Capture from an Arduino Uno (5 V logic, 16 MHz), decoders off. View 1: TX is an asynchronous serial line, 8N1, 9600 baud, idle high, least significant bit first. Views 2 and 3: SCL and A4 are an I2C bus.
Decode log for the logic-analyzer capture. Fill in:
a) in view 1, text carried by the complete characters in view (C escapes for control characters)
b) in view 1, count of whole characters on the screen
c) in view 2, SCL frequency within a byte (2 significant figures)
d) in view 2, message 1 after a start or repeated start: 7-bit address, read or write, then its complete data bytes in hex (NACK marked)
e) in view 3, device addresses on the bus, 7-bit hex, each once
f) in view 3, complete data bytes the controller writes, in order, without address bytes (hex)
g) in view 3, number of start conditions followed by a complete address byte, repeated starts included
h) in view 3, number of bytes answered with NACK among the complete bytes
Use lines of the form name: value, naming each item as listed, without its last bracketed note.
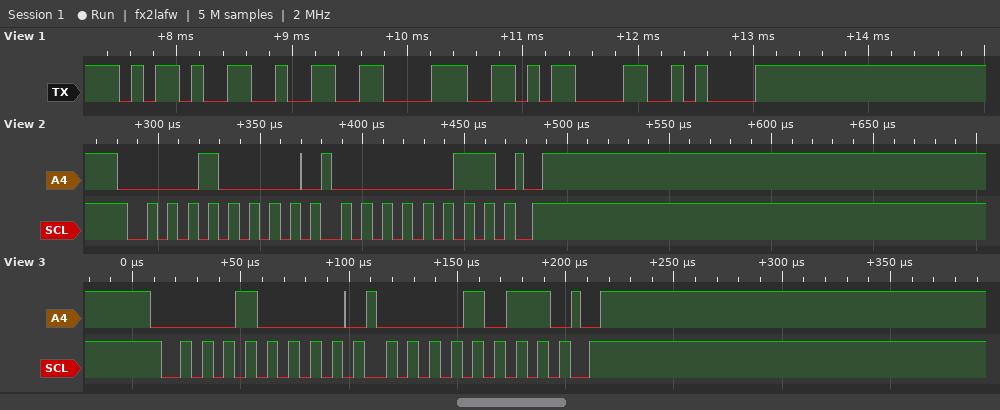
in view 1, text carried by the complete characters in view: "-28\r\n"
in view 1, count of whole characters on the screen: 5
in view 2, SCL frequency within a byte: 100 kHz
in view 2, message 1 after a start or repeated start: 7-bit address, read or write, then its complete data bytes in hex: 0x08 write: 03
in view 3, device addresses on the bus, 7-bit hex, each once: 0x08
in view 3, complete data bytes the controller writes, in order, without address bytes: 0B
in view 3, number of start conditions followed by a complete address byte, repeated starts included: 1
in view 3, number of bytes answered with NACK among the complete bytes: 0
